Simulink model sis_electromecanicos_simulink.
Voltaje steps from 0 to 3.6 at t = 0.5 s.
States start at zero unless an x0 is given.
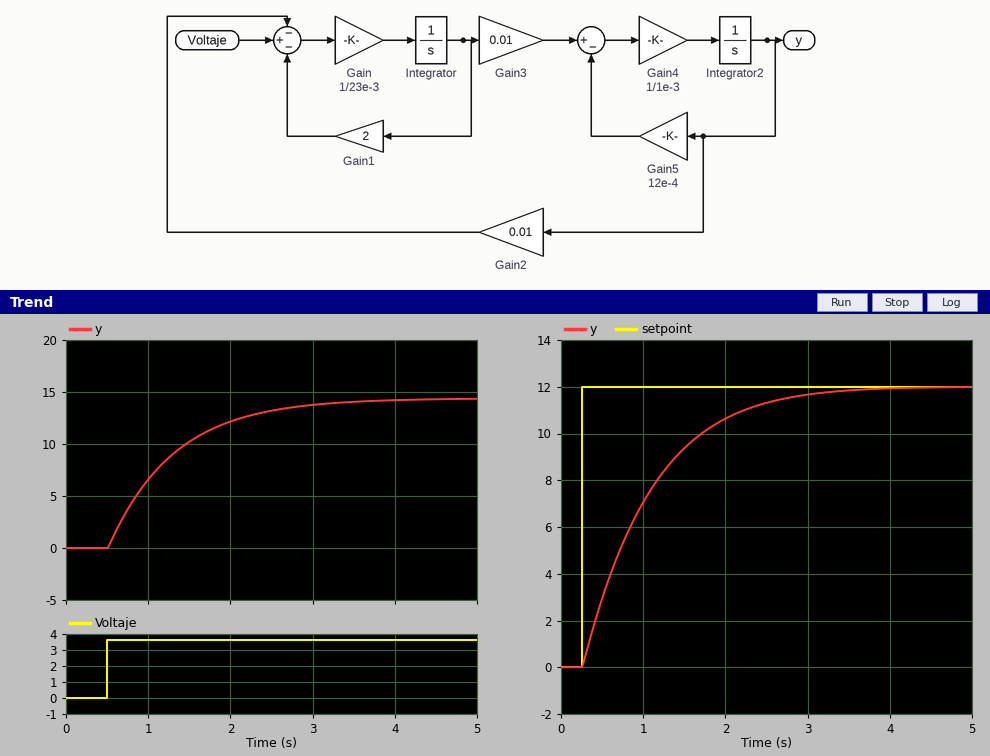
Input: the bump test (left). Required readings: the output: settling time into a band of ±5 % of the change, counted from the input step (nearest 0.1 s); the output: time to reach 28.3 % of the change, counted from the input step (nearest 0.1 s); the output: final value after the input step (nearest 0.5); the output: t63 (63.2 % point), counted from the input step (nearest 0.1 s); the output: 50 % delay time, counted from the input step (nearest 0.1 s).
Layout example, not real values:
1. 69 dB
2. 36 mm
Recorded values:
1. 2.4 s
2. 0.3 s
3. 14.5
4. 0.8 s
5. 0.6 s
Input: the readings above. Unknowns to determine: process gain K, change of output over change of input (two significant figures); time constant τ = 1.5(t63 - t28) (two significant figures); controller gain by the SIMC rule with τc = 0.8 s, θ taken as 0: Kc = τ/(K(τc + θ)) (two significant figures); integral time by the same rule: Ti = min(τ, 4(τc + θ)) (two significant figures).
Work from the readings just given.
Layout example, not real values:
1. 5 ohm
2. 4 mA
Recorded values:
1. 4.0
2. 0.75 s
3. 0.23
4. 0.75 s
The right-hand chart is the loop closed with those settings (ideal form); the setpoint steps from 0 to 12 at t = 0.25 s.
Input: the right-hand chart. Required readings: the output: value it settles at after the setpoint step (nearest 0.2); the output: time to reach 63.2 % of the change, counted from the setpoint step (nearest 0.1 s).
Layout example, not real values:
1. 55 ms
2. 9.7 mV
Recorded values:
1. 12.0
2. 0.8 s
